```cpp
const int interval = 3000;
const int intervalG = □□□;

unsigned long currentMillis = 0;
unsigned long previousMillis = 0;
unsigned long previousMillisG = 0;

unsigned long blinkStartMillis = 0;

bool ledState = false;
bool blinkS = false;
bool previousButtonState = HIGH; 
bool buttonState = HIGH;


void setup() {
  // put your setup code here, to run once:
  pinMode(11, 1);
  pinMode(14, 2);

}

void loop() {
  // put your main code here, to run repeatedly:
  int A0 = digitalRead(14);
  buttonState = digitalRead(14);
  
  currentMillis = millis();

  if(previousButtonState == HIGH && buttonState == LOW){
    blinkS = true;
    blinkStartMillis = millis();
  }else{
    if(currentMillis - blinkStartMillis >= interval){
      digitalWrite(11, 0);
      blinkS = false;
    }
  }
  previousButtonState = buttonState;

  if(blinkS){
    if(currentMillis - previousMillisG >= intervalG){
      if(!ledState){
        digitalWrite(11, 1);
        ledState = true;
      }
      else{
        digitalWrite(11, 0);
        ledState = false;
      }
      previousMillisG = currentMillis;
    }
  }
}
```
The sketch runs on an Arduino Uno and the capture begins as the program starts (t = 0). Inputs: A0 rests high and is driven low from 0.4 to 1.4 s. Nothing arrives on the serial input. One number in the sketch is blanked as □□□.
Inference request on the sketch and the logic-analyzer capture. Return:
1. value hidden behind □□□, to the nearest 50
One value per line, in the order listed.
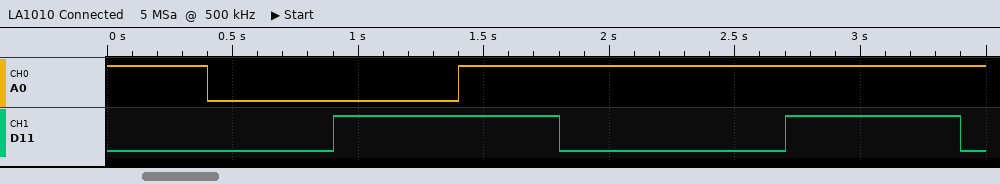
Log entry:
900
